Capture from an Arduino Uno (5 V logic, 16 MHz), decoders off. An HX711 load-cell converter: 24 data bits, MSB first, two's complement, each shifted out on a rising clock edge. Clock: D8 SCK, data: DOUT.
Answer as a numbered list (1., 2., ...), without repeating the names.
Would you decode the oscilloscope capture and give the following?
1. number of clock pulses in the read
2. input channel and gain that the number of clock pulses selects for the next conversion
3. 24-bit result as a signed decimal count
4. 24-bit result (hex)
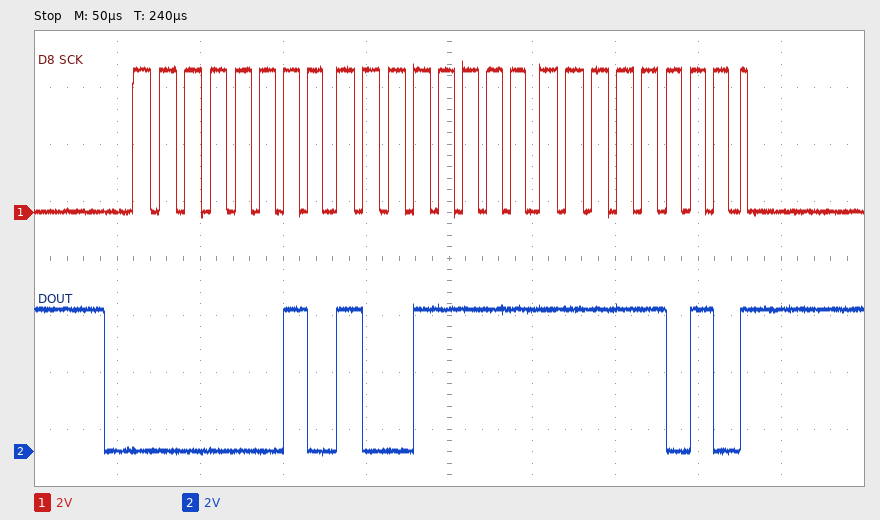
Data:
1. 25
2. channel A, gain 128
3. 172026
4. 0x029FFA
